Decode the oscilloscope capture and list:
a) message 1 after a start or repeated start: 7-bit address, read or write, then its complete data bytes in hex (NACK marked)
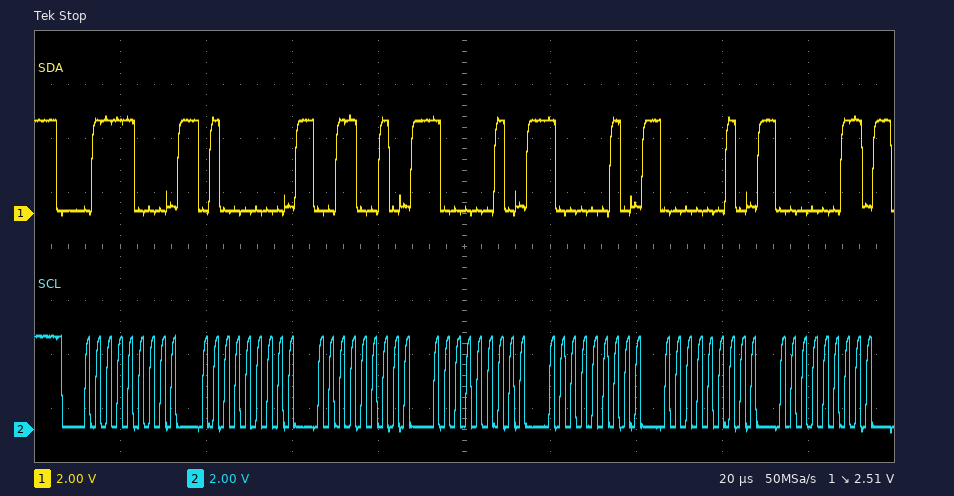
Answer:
0x3C write: 40 32 82 82 02 03
